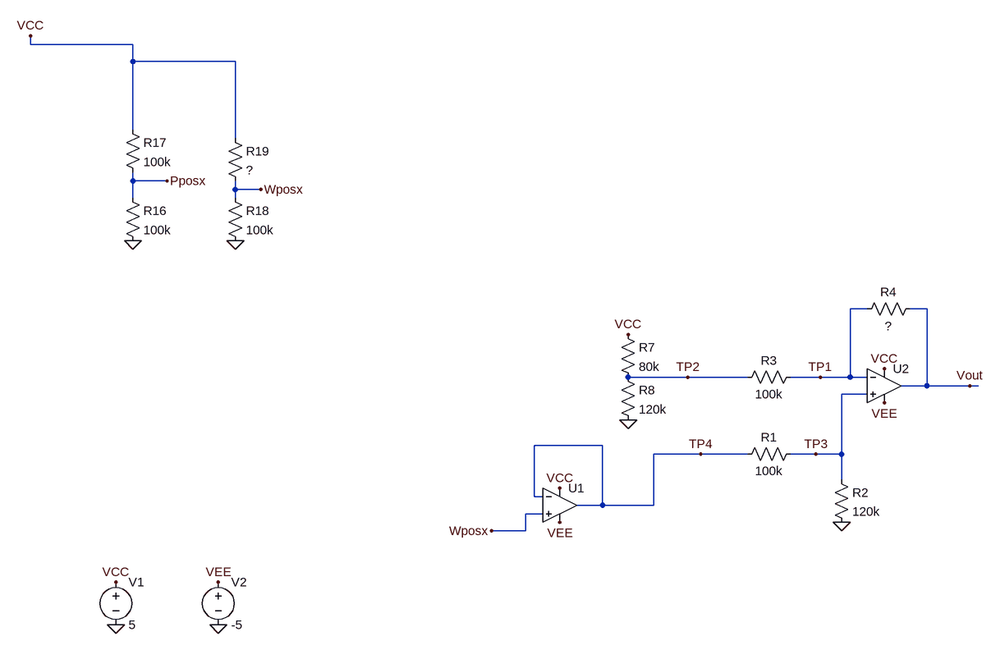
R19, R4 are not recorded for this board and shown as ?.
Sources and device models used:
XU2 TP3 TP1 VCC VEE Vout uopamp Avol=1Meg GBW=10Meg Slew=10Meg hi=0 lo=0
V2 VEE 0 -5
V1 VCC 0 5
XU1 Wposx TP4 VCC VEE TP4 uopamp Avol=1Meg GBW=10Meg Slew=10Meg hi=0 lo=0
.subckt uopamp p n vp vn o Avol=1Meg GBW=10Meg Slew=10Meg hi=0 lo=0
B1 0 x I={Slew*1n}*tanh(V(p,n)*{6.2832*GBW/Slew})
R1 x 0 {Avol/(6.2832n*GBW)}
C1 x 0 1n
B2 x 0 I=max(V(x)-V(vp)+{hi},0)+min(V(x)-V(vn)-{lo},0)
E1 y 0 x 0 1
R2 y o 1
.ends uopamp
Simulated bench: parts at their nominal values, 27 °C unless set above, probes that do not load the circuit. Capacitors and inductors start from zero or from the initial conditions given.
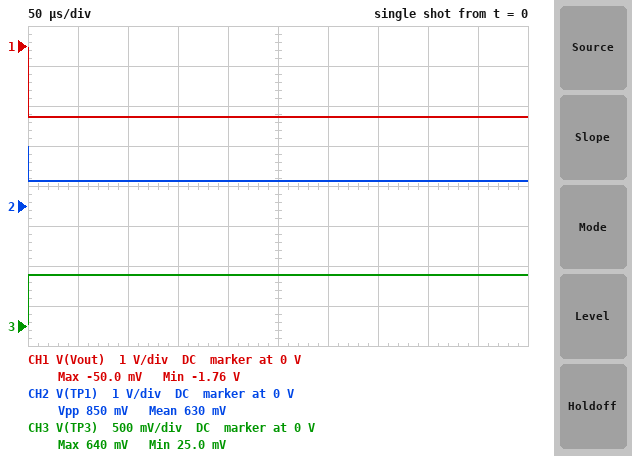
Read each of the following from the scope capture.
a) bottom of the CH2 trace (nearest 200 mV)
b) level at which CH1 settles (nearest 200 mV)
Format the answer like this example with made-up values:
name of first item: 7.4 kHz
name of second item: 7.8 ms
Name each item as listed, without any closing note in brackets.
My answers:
bottom of the CH2 trace: 600 mV
level at which CH1 settles: -1.8 V
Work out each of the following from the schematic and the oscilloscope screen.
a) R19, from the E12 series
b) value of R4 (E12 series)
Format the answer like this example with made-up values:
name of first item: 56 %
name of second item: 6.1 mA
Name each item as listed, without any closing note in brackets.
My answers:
R19, from the E12 series: 330 kΩ
value of R4: 150 kΩ
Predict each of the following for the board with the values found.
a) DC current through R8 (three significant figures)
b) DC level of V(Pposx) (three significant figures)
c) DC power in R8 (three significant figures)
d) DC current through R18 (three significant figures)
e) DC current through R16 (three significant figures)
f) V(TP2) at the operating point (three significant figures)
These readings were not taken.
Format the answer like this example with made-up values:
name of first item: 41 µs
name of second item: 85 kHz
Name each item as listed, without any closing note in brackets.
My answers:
DC current through R8: 18.6 µA
DC level of V(Pposx): 2.50 V
DC power in R8: 41.5 µW
DC current through R18: 11.6 µA
DC current through R16: 25.0 µA
V(TP2) at the operating point: 2.23 V
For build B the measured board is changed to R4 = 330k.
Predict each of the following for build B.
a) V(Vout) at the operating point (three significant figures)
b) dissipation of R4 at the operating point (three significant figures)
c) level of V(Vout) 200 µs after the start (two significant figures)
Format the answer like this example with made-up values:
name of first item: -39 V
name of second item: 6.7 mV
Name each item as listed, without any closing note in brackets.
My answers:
V(Vout) at the operating point: -4.64 V
dissipation of R4 at the operating point: 84.3 µW
level of V(Vout) 200 µs after the start: -4.6 V
